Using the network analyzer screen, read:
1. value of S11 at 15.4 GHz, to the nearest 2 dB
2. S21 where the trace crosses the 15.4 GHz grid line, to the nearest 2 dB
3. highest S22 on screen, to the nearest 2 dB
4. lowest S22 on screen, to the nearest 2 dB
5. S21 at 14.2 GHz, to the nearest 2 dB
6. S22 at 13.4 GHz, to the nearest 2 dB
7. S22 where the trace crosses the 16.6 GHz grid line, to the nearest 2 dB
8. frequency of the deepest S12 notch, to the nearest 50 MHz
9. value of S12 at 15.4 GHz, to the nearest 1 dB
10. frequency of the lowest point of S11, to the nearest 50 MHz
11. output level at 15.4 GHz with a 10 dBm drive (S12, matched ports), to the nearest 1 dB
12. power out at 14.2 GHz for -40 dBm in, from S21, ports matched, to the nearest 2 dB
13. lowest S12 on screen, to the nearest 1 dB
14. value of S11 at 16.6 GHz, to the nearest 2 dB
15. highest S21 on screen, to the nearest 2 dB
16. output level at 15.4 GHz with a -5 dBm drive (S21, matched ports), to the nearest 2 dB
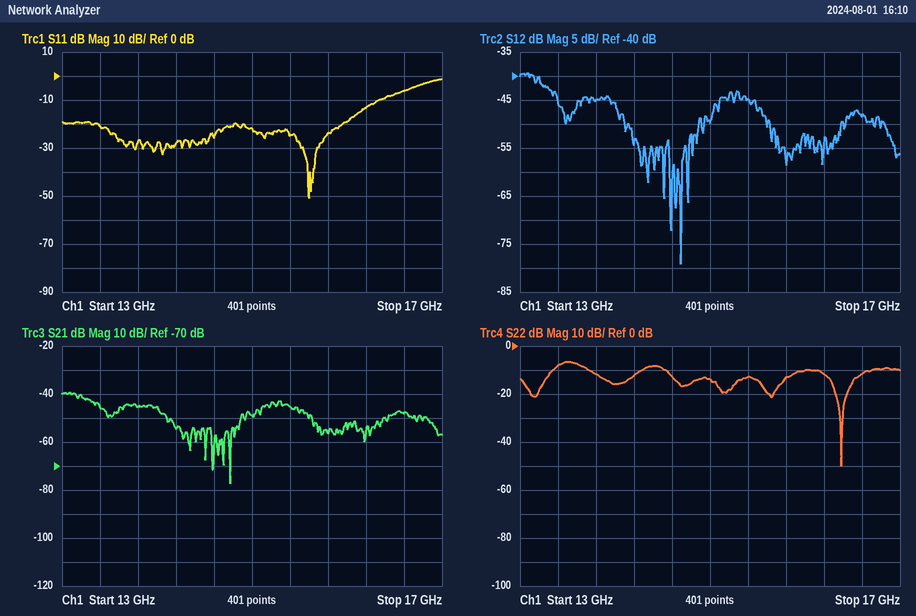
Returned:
-24 dB
-46 dB
-6 dB
-50 dB
-54 dB
-8 dB
-12 dB
14.70 GHz
-45 dB
15.60 GHz
-35 dBm
-94 dBm
-79 dB
-6 dB
-40 dB
-50 dBm
